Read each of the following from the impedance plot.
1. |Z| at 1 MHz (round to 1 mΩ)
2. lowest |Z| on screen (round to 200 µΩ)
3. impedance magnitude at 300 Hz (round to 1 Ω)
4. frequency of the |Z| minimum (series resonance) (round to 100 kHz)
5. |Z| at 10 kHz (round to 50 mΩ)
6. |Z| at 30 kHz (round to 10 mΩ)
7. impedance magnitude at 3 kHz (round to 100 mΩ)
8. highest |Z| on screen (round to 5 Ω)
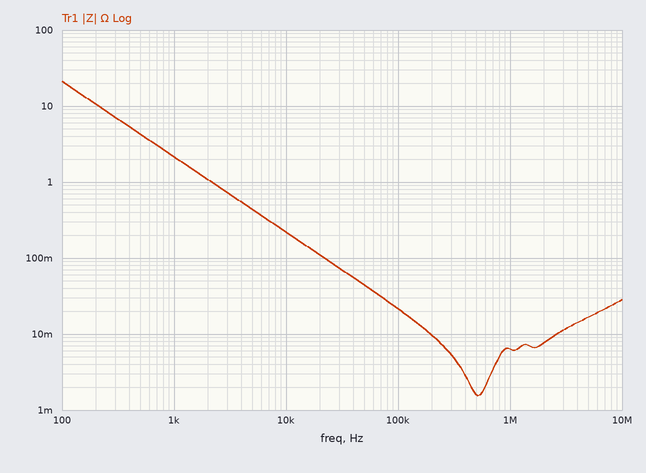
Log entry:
6 mΩ
1.6 mΩ
7 Ω
500 kHz
200 mΩ
70 mΩ
700 mΩ
20 Ω
